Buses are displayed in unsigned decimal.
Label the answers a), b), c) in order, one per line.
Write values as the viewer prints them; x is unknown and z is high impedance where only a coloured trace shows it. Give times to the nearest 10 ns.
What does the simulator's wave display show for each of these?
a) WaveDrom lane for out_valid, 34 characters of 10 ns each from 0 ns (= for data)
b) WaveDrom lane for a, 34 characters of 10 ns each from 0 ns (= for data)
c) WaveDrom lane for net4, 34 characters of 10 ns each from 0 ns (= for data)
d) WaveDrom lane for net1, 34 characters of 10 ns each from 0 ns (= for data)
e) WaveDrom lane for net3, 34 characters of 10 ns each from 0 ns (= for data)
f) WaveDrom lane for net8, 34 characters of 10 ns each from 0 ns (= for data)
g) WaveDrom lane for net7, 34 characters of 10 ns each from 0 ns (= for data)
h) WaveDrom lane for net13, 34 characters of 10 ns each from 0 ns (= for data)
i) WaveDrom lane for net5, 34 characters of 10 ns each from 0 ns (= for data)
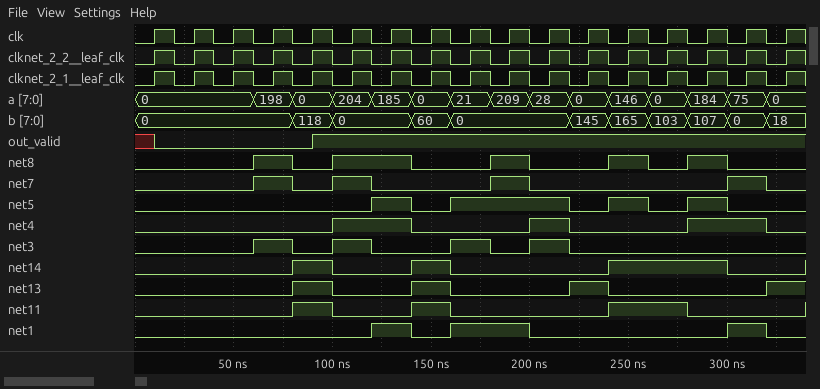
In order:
a) {name: 'out_valid', wave: 'x0.......1........................'}
b) {name: 'a', wave: '=.....=.=.=.=.=.=.=.=.=.=.=.=.=.=.', data: '0 198 0 204 185 0 21 209 28 0 146 0 184 75 0'}
c) {name: 'net4', wave: '0.........1...0.....1.0.....1...0.'}
d) {name: 'net1', wave: '0...........1.0.1...0.........1.0.'}
e) {name: 'net3', wave: '0.....1.0.1.0...1.0.1.0...........'}
f) {name: 'net8', wave: '0.....1.0.1...0...1.0...1.0.1.0...'}
g) {name: 'net7', wave: '0.....1.0.1.0.....1.0.........1.0.'}
h) {name: 'net13', wave: '0.......1.0...1.0.....1.0.......1.'}
i) {name: 'net5', wave: '0...........1.0.1.....0.1.0.1.0...'}
